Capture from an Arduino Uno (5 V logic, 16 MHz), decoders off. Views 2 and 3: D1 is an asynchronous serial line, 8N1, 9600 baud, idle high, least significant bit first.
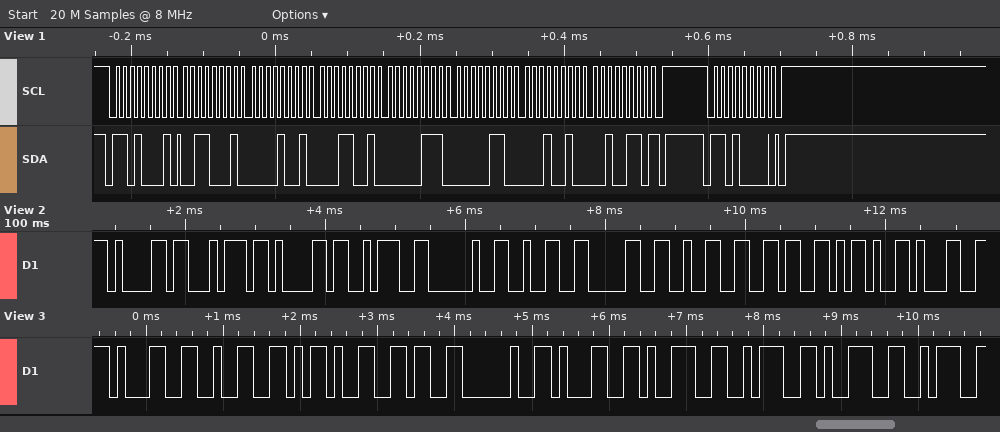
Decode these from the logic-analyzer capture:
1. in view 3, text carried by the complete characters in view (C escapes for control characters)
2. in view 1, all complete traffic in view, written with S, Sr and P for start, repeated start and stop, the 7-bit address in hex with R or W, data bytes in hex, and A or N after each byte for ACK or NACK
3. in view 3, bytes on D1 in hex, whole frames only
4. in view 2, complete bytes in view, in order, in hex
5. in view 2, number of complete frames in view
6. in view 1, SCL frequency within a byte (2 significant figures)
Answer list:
"12-6 19:9:"
S 68R A 31 A 09 A 19 A 07 A 06 A 12 A 26 N P S 68W A P
31 32 2D 36 20 31 39 3A 39 3A
61 74 61 3A 20 32 30 32 36 2D 31
11
100 kHz
